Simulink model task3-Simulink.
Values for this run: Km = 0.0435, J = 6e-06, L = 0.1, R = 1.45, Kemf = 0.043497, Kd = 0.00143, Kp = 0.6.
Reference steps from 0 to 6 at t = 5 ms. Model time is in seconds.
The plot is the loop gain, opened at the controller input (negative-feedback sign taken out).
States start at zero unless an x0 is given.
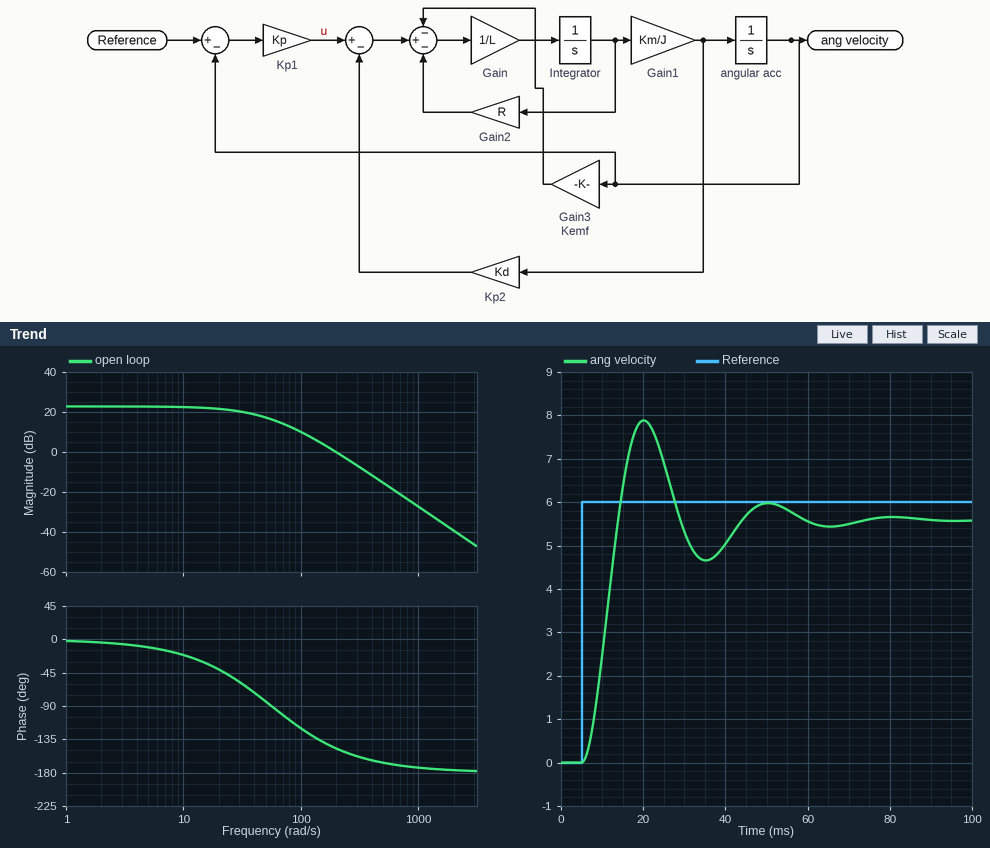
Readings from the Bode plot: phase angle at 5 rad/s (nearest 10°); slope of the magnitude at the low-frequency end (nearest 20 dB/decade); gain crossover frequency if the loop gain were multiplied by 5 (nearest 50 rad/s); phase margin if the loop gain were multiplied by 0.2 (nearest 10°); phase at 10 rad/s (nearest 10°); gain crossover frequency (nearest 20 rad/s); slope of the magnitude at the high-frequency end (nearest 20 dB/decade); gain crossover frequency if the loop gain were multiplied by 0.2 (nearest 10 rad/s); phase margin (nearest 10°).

-10°
0 dB/decade
450 rad/s
80°
-20°
200 rad/s
-40 dB/decade
70 rad/s
30°
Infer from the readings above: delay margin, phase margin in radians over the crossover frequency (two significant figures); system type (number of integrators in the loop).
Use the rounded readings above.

0.0026 s
0
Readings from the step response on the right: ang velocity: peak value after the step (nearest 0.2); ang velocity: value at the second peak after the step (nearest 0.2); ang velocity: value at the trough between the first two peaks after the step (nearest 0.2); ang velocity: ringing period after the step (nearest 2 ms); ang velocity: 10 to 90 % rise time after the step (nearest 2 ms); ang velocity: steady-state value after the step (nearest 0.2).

7.8
6.0
4.6
30 ms
6 ms
5.6
